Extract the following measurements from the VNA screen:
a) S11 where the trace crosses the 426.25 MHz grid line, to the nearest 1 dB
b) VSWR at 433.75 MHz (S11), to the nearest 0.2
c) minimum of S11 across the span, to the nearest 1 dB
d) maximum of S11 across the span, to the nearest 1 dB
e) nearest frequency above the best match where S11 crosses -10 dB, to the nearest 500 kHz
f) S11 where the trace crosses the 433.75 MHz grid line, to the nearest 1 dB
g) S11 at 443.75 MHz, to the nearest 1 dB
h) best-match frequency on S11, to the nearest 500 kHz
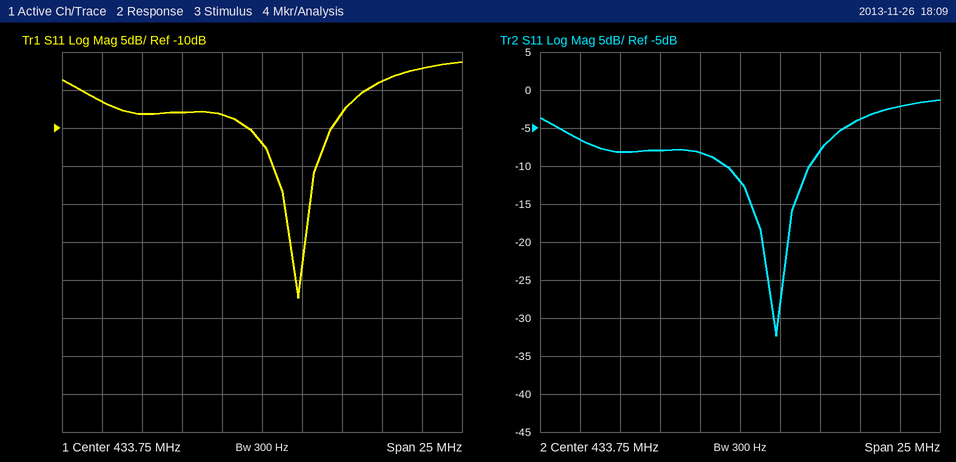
-8 dB
1.6
-32 dB
-1 dB
438.0 MHz
-12 dB
-2 dB
436.0 MHz
